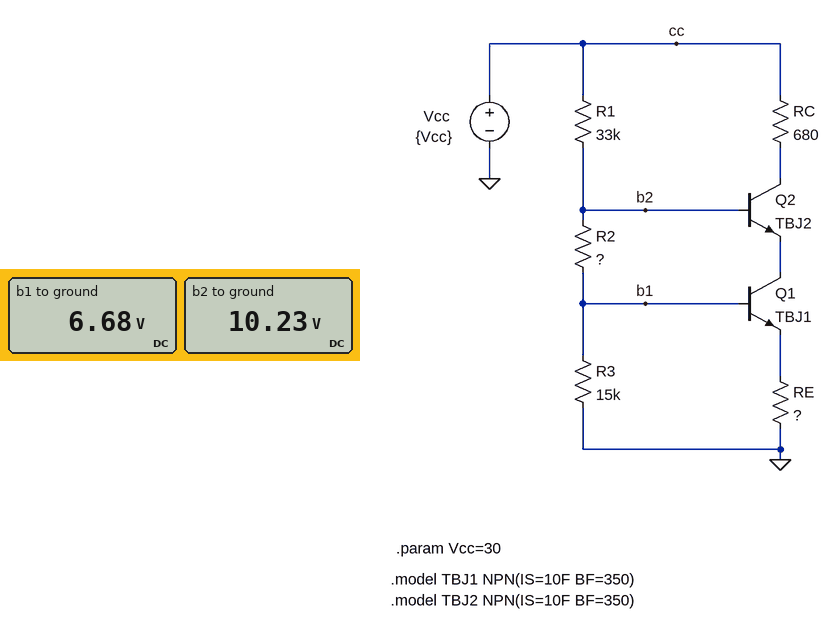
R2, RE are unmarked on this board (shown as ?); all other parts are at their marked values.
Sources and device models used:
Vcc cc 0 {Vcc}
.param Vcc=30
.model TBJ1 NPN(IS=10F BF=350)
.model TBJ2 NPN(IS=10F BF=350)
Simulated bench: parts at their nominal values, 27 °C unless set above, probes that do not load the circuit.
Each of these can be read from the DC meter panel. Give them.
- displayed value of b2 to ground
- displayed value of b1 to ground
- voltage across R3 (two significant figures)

10.23 V
6.68 V
6.7 V
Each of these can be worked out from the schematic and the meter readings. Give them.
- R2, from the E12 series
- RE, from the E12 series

6.8 kΩ
220 Ω
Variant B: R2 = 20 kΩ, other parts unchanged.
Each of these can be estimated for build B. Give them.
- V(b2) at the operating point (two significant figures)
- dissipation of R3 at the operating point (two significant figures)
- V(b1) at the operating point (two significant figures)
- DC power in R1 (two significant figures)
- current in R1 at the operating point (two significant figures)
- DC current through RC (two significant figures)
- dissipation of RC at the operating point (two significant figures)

14 V
2.0 mW
5.5 V
7.8 mW
490 µA
21 mA
310 mW
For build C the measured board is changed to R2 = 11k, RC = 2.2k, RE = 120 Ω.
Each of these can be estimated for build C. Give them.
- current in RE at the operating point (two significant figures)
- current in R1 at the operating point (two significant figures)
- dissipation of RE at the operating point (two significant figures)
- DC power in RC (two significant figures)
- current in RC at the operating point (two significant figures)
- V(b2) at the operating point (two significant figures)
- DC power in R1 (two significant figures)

13 mA
780 µA
19 mW
320 mW
12 mA
4.3 V
20 mW
